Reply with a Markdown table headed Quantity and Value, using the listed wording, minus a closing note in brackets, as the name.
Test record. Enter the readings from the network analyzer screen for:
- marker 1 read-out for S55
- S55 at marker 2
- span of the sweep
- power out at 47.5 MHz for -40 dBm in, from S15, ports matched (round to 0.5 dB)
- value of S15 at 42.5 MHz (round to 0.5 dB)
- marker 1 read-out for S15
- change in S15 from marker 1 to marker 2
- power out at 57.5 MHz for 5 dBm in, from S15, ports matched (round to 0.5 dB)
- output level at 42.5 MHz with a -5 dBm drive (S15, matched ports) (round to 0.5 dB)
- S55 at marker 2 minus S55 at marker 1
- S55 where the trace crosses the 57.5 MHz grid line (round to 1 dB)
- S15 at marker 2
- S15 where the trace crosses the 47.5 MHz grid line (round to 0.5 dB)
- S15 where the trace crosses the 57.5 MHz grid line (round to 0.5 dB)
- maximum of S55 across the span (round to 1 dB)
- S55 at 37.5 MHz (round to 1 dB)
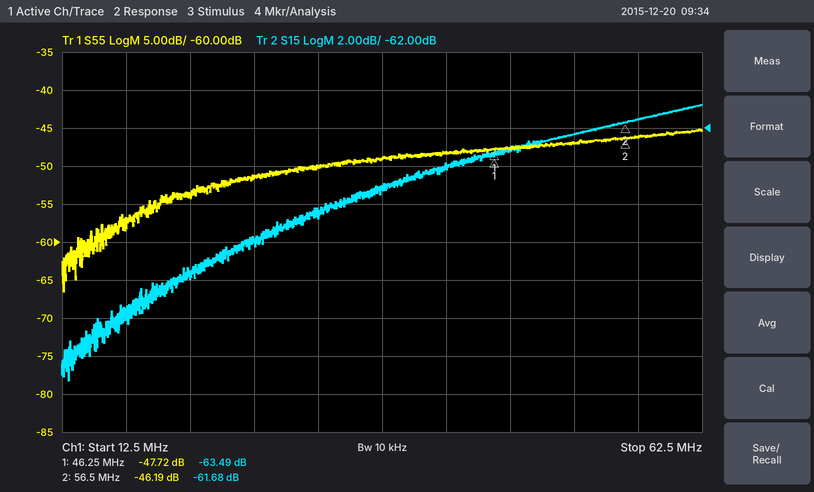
| Quantity | Value |
|---|---|
| marker 1 read-out for S55 | -47.72 dB |
| S55 at marker 2 | -46.19 dB |
| span of the sweep | 50 MHz |
| power out at 47.5 MHz for -40 dBm in, from S15, ports matched | -103.0 dBm |
| value of S15 at 42.5 MHz | -64.0 dB |
| marker 1 read-out for S15 | -63.49 dB |
| change in S15 from marker 1 to marker 2 | 1.81 dB |
| power out at 57.5 MHz for 5 dBm in, from S15, ports matched | -56.5 dBm |
| output level at 42.5 MHz with a -5 dBm drive (S15, matched ports) | -69.0 dBm |
| S55 at marker 2 minus S55 at marker 1 | 1.53 dB |
| S55 where the trace crosses the 57.5 MHz grid line | -46 dB |
| S15 at marker 2 | -61.68 dB |
| S15 where the trace crosses the 47.5 MHz grid line | -63.0 dB |
| S15 where the trace crosses the 57.5 MHz grid line | -61.5 dB |
| maximum of S55 across the span | -45 dB |
| S55 at 37.5 MHz | -49 dB |
